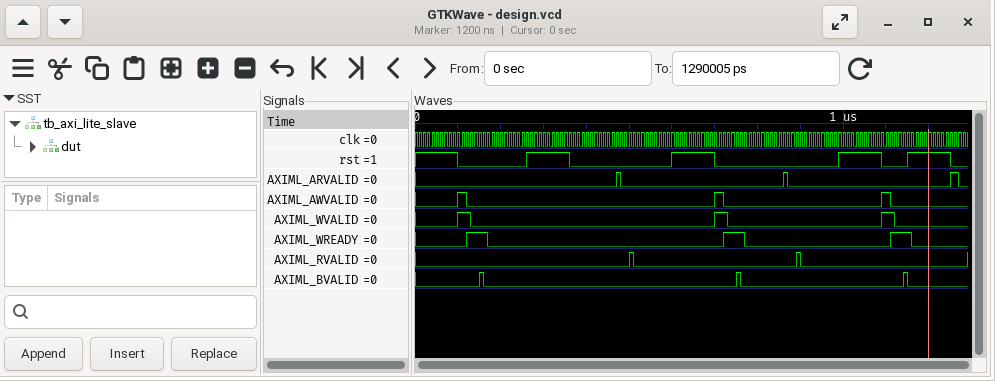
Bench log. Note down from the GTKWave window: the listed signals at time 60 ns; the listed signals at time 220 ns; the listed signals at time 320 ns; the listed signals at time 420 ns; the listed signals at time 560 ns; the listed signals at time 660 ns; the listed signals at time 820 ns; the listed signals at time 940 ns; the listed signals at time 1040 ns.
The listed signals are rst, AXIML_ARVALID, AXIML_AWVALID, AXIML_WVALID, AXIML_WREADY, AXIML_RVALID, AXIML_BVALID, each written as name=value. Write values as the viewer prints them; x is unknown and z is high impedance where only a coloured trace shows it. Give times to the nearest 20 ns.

rst=1, AXIML_ARVALID=0, AXIML_AWVALID=0, AXIML_WVALID=0, AXIML_WREADY=0, AXIML_RVALID=0, AXIML_BVALID=0
rst=0, AXIML_ARVALID=0, AXIML_AWVALID=0, AXIML_WVALID=0, AXIML_WREADY=0, AXIML_RVALID=0, AXIML_BVALID=0
rst=1, AXIML_ARVALID=0, AXIML_AWVALID=0, AXIML_WVALID=0, AXIML_WREADY=0, AXIML_RVALID=0, AXIML_BVALID=0
rst=0, AXIML_ARVALID=0, AXIML_AWVALID=0, AXIML_WVALID=0, AXIML_WREADY=0, AXIML_RVALID=0, AXIML_BVALID=0
rst=0, AXIML_ARVALID=0, AXIML_AWVALID=0, AXIML_WVALID=0, AXIML_WREADY=0, AXIML_RVALID=0, AXIML_BVALID=0
rst=1, AXIML_ARVALID=0, AXIML_AWVALID=0, AXIML_WVALID=0, AXIML_WREADY=0, AXIML_RVALID=0, AXIML_BVALID=0
rst=0, AXIML_ARVALID=0, AXIML_AWVALID=0, AXIML_WVALID=0, AXIML_WREADY=0, AXIML_RVALID=0, AXIML_BVALID=0
rst=0, AXIML_ARVALID=0, AXIML_AWVALID=0, AXIML_WVALID=0, AXIML_WREADY=0, AXIML_RVALID=0, AXIML_BVALID=0
rst=1, AXIML_ARVALID=0, AXIML_AWVALID=0, AXIML_WVALID=0, AXIML_WREADY=0, AXIML_RVALID=0, AXIML_BVALID=0
